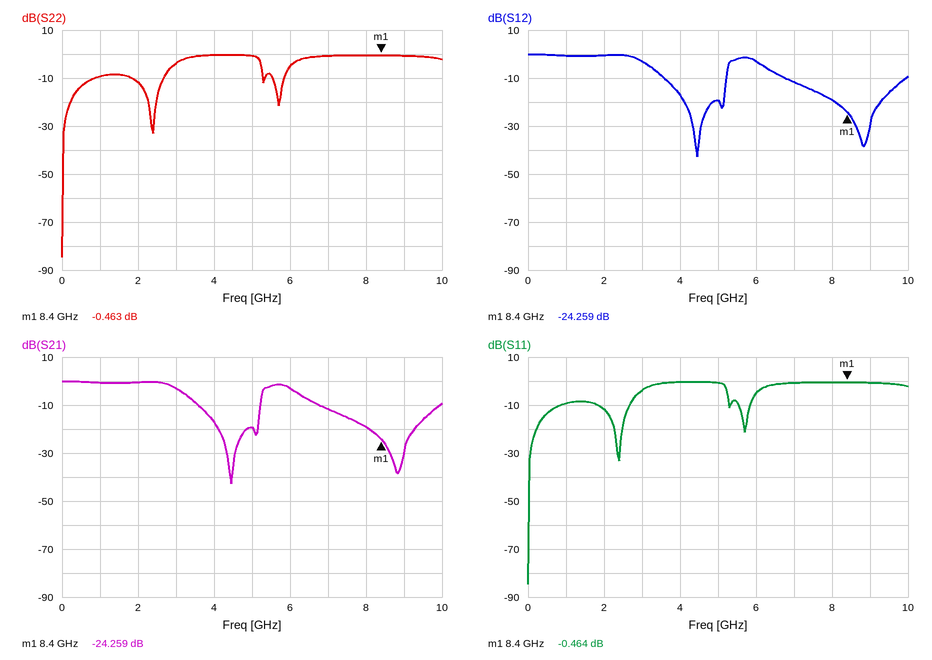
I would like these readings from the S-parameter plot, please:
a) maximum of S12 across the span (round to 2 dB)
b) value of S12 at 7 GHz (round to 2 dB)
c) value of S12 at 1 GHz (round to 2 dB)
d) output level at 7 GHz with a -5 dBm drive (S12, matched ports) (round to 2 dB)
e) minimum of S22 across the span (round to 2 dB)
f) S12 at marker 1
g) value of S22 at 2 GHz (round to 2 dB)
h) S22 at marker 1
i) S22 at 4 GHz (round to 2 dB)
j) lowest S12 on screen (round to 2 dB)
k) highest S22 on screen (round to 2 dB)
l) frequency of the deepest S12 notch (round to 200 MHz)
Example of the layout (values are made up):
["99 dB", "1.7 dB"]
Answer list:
["0 dB", "-12 dB", "0 dB", "-16 dBm", "-84 dB", "-24.259 dB", "-12 dB", "-0.463 dB", "0 dB", "-42 dB", "0 dB", "4.4 GHz"]
